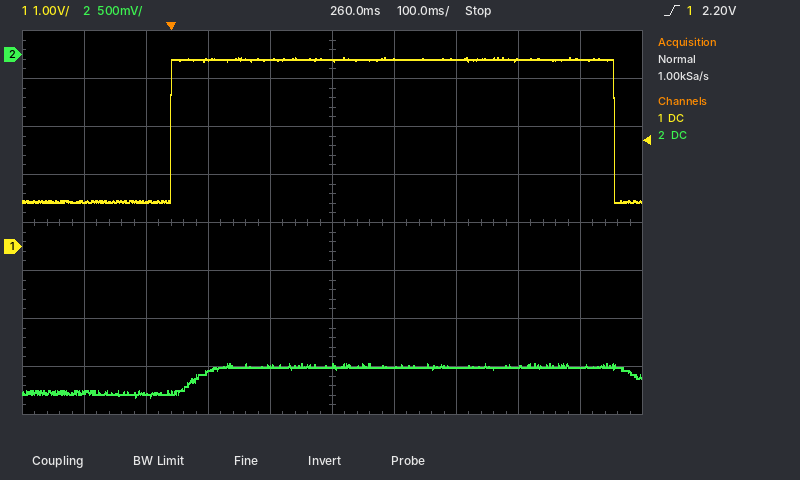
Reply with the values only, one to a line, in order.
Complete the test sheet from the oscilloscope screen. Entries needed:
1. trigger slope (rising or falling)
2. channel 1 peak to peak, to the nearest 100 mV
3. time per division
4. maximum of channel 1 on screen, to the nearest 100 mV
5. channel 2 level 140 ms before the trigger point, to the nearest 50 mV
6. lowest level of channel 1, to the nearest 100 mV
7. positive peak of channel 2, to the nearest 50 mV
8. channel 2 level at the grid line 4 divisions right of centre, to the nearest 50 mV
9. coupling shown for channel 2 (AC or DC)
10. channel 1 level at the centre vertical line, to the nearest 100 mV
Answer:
rising
3.0 V
100 ms
3.9 V
-3.50 V
900 mV
-3.20 V
-3.25 V
DC
3.9 V
